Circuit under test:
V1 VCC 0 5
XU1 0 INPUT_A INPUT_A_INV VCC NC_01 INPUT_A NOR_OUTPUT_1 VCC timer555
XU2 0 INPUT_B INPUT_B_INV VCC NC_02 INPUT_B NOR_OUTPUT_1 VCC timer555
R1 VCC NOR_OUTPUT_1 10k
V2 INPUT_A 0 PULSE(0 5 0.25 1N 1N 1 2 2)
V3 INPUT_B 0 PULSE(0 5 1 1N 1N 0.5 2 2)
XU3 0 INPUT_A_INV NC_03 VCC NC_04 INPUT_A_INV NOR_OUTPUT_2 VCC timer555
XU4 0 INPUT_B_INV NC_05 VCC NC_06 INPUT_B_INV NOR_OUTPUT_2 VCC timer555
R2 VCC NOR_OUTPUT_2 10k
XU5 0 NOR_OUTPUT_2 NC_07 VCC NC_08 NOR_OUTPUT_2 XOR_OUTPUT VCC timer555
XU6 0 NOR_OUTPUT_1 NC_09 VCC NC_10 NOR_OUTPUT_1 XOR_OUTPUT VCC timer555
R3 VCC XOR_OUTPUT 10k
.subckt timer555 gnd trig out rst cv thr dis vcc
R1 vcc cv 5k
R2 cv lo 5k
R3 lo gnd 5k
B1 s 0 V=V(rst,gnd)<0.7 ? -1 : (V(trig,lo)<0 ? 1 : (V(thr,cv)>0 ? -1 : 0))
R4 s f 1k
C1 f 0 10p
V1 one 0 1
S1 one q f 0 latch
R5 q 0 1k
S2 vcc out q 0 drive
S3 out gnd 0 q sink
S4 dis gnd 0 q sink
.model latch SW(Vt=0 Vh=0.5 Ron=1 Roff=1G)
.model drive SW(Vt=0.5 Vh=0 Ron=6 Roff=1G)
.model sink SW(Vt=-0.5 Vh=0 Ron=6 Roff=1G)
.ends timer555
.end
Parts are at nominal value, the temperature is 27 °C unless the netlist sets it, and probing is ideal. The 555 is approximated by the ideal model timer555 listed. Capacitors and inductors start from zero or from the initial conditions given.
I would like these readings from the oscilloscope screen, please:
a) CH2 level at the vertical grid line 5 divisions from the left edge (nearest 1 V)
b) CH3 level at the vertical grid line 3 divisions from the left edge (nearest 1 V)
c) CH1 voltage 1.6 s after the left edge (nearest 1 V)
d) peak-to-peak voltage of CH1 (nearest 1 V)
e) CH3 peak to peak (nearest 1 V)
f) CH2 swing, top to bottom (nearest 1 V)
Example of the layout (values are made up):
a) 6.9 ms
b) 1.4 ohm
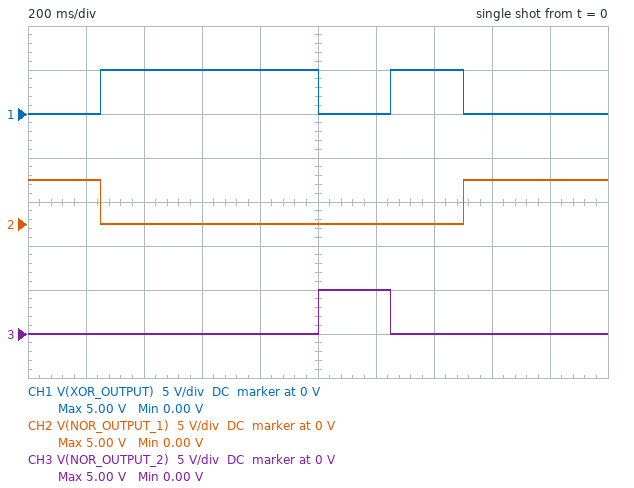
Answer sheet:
a) 0 V
b) 0 V
c) 0 V
d) 5 V
e) 5 V
f) 5 V
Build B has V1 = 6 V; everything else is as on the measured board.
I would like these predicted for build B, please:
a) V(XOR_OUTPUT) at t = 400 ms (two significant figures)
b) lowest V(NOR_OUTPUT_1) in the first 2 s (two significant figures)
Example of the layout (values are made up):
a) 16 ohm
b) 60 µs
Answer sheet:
a) 6.0 V
b) 1.8 mV
